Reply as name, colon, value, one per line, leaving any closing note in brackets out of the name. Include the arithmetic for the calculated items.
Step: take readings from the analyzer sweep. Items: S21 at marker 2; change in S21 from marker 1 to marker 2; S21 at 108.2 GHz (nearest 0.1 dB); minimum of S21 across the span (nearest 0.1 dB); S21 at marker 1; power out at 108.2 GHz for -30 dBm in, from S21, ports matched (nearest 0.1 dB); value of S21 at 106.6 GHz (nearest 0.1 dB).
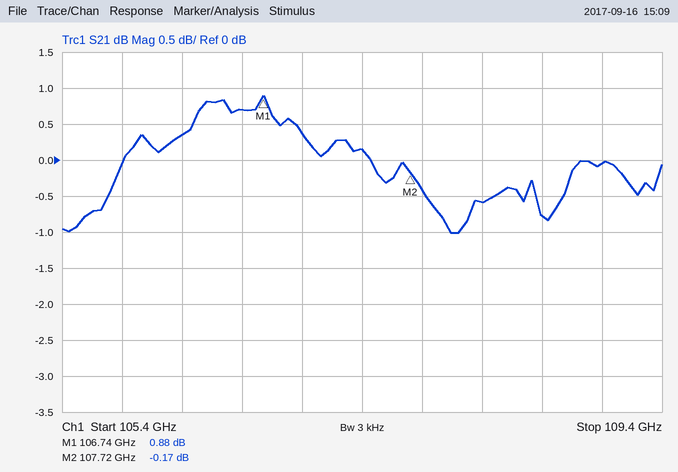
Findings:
S21 at marker 2: -0.17 dB
change in S21 from marker 1 to marker 2: -0.17 − (0.88) = -1.05 dB
S21 at 108.2 GHz: -0.6 dB
minimum of S21 across the span: -1.0 dB
S21 at marker 1: 0.88 dB
power out at 108.2 GHz for -30 dBm in, from S21, ports matched: -30 dBm + (-0.6 dB) = -30.6 dBm
value of S21 at 106.6 GHz: 0.7 dB
